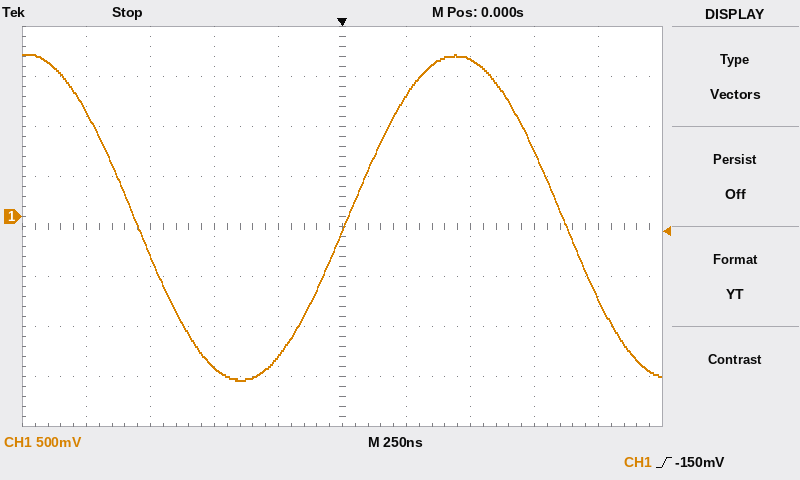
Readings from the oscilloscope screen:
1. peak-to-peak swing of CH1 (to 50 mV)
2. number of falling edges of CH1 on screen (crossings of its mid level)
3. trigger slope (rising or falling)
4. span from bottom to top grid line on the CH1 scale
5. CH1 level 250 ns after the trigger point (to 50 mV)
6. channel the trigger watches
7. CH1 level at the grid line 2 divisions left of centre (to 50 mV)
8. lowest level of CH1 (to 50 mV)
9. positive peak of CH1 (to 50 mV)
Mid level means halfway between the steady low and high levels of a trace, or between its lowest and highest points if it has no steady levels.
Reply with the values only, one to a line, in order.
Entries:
3.25 V
2
rising
4 V
1.20 V
CH1
-1.50 V
-1.65 V
1.60 V
